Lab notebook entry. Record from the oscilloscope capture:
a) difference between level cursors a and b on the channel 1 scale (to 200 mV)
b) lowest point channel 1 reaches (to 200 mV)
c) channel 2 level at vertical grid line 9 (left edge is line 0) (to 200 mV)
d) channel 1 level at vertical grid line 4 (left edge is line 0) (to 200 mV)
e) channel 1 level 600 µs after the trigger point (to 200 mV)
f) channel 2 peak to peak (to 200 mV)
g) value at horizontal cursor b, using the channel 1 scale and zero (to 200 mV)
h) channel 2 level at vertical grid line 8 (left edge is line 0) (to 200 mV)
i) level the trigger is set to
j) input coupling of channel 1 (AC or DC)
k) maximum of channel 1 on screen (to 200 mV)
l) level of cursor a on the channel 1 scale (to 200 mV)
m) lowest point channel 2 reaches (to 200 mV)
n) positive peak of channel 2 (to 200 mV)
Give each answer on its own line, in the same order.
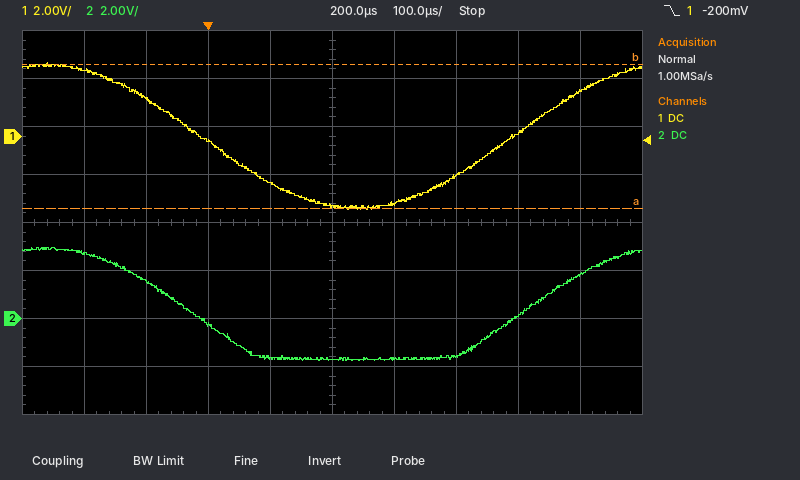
6.0 V
-3.0 V
1.8 V
-2.0 V
1.8 V
4.8 V
3.0 V
200 mV
-200 mV
DC
3.0 V
-3.0 V
-1.8 V
3.0 V
